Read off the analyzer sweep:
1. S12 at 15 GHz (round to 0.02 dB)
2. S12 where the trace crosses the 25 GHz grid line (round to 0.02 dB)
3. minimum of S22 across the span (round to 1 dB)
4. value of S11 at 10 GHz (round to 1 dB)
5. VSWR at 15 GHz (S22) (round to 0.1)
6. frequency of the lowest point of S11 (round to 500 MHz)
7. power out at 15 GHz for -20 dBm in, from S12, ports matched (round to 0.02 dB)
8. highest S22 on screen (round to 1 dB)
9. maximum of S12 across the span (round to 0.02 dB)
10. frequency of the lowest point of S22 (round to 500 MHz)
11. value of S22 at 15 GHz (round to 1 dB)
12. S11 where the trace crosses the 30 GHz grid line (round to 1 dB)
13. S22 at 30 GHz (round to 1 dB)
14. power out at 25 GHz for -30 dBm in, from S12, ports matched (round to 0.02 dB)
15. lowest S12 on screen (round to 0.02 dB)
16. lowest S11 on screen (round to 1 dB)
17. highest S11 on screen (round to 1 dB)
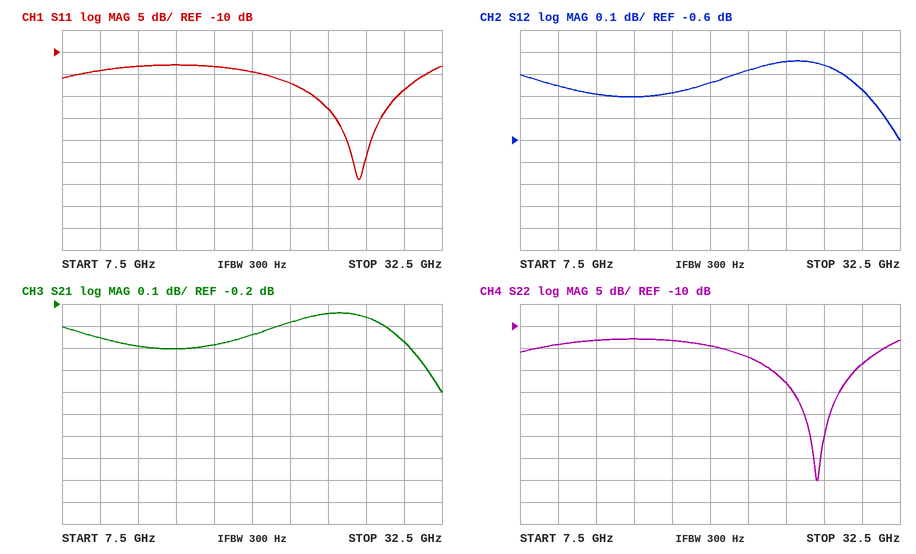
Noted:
-0.40 dB
-0.24 dB
-45 dB
-14 dB
1.6
27.0 GHz
-20.40 dBm
-13 dB
-0.24 dB
27.0 GHz
-13 dB
-19 dB
-19 dB
-30.24 dBm
-0.60 dB
-39 dB
-13 dB
